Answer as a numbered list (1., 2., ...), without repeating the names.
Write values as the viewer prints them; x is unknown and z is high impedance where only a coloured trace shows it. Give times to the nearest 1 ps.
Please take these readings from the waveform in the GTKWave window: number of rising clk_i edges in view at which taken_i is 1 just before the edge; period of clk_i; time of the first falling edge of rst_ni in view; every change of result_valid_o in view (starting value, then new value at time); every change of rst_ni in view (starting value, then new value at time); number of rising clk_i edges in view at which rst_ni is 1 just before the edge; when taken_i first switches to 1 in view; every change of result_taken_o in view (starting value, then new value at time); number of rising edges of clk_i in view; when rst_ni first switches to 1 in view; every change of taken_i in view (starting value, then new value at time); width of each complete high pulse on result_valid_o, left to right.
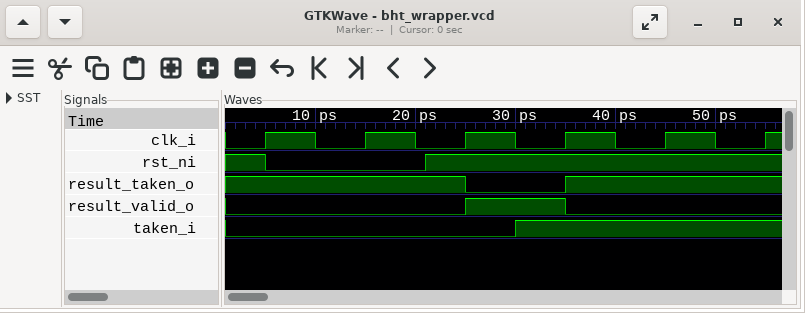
1. 3
2. 10 ps
3. 5 ps
4. 0, 1 at 25 ps, 0 at 35 ps
5. 1, 0 at 5 ps, 1 at 21 ps
6. 5
7. 30 ps
8. 1, 0 at 25 ps, 1 at 35 ps
9. 6
10. 21 ps
11. 0, 1 at 30 ps
12. 10 ps
